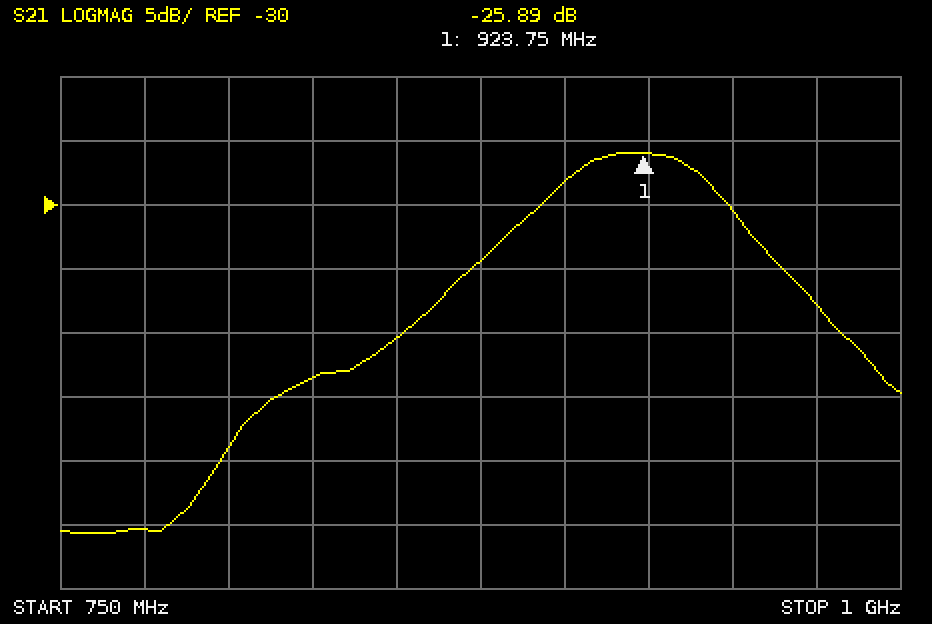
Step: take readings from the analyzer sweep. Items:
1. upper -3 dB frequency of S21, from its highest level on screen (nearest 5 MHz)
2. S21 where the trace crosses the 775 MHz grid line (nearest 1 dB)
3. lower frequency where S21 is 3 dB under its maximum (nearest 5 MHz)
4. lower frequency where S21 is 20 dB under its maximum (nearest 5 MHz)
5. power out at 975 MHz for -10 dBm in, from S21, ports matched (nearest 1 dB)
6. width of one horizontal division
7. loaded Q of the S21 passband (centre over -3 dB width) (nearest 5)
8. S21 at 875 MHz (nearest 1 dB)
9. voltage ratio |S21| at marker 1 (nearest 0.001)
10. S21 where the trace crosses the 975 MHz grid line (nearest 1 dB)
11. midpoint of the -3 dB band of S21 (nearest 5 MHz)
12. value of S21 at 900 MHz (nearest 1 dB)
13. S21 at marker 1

945 MHz
-55 dB
895 MHz
810 MHz
-48 dBm
25 MHz
20
-34 dB
0.051
-38 dB
920 MHz
-28 dB
-25.89 dB
